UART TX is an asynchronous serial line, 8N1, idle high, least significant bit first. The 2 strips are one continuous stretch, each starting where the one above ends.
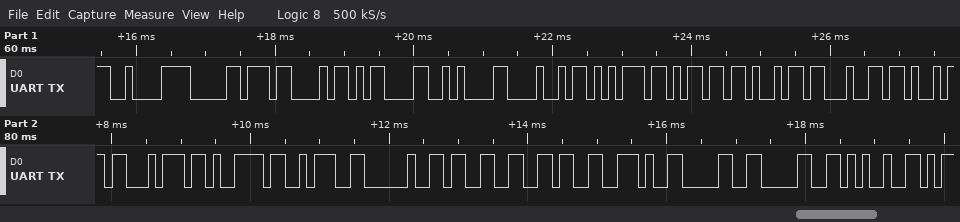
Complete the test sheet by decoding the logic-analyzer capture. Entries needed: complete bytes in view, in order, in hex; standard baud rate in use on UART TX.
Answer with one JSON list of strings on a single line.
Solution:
["C2 B0 43 0D 0A 48 75 6D 69 64 69 74 79 3A 20 33 36 2E 30 30 25", "9600 baud"]
